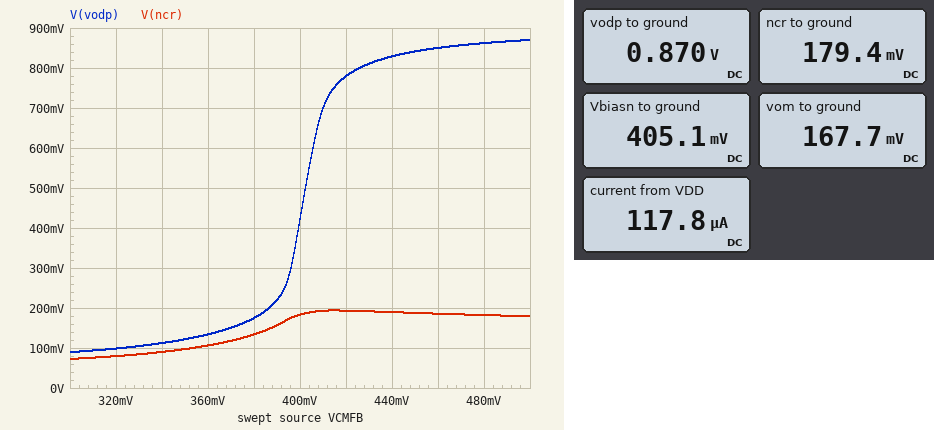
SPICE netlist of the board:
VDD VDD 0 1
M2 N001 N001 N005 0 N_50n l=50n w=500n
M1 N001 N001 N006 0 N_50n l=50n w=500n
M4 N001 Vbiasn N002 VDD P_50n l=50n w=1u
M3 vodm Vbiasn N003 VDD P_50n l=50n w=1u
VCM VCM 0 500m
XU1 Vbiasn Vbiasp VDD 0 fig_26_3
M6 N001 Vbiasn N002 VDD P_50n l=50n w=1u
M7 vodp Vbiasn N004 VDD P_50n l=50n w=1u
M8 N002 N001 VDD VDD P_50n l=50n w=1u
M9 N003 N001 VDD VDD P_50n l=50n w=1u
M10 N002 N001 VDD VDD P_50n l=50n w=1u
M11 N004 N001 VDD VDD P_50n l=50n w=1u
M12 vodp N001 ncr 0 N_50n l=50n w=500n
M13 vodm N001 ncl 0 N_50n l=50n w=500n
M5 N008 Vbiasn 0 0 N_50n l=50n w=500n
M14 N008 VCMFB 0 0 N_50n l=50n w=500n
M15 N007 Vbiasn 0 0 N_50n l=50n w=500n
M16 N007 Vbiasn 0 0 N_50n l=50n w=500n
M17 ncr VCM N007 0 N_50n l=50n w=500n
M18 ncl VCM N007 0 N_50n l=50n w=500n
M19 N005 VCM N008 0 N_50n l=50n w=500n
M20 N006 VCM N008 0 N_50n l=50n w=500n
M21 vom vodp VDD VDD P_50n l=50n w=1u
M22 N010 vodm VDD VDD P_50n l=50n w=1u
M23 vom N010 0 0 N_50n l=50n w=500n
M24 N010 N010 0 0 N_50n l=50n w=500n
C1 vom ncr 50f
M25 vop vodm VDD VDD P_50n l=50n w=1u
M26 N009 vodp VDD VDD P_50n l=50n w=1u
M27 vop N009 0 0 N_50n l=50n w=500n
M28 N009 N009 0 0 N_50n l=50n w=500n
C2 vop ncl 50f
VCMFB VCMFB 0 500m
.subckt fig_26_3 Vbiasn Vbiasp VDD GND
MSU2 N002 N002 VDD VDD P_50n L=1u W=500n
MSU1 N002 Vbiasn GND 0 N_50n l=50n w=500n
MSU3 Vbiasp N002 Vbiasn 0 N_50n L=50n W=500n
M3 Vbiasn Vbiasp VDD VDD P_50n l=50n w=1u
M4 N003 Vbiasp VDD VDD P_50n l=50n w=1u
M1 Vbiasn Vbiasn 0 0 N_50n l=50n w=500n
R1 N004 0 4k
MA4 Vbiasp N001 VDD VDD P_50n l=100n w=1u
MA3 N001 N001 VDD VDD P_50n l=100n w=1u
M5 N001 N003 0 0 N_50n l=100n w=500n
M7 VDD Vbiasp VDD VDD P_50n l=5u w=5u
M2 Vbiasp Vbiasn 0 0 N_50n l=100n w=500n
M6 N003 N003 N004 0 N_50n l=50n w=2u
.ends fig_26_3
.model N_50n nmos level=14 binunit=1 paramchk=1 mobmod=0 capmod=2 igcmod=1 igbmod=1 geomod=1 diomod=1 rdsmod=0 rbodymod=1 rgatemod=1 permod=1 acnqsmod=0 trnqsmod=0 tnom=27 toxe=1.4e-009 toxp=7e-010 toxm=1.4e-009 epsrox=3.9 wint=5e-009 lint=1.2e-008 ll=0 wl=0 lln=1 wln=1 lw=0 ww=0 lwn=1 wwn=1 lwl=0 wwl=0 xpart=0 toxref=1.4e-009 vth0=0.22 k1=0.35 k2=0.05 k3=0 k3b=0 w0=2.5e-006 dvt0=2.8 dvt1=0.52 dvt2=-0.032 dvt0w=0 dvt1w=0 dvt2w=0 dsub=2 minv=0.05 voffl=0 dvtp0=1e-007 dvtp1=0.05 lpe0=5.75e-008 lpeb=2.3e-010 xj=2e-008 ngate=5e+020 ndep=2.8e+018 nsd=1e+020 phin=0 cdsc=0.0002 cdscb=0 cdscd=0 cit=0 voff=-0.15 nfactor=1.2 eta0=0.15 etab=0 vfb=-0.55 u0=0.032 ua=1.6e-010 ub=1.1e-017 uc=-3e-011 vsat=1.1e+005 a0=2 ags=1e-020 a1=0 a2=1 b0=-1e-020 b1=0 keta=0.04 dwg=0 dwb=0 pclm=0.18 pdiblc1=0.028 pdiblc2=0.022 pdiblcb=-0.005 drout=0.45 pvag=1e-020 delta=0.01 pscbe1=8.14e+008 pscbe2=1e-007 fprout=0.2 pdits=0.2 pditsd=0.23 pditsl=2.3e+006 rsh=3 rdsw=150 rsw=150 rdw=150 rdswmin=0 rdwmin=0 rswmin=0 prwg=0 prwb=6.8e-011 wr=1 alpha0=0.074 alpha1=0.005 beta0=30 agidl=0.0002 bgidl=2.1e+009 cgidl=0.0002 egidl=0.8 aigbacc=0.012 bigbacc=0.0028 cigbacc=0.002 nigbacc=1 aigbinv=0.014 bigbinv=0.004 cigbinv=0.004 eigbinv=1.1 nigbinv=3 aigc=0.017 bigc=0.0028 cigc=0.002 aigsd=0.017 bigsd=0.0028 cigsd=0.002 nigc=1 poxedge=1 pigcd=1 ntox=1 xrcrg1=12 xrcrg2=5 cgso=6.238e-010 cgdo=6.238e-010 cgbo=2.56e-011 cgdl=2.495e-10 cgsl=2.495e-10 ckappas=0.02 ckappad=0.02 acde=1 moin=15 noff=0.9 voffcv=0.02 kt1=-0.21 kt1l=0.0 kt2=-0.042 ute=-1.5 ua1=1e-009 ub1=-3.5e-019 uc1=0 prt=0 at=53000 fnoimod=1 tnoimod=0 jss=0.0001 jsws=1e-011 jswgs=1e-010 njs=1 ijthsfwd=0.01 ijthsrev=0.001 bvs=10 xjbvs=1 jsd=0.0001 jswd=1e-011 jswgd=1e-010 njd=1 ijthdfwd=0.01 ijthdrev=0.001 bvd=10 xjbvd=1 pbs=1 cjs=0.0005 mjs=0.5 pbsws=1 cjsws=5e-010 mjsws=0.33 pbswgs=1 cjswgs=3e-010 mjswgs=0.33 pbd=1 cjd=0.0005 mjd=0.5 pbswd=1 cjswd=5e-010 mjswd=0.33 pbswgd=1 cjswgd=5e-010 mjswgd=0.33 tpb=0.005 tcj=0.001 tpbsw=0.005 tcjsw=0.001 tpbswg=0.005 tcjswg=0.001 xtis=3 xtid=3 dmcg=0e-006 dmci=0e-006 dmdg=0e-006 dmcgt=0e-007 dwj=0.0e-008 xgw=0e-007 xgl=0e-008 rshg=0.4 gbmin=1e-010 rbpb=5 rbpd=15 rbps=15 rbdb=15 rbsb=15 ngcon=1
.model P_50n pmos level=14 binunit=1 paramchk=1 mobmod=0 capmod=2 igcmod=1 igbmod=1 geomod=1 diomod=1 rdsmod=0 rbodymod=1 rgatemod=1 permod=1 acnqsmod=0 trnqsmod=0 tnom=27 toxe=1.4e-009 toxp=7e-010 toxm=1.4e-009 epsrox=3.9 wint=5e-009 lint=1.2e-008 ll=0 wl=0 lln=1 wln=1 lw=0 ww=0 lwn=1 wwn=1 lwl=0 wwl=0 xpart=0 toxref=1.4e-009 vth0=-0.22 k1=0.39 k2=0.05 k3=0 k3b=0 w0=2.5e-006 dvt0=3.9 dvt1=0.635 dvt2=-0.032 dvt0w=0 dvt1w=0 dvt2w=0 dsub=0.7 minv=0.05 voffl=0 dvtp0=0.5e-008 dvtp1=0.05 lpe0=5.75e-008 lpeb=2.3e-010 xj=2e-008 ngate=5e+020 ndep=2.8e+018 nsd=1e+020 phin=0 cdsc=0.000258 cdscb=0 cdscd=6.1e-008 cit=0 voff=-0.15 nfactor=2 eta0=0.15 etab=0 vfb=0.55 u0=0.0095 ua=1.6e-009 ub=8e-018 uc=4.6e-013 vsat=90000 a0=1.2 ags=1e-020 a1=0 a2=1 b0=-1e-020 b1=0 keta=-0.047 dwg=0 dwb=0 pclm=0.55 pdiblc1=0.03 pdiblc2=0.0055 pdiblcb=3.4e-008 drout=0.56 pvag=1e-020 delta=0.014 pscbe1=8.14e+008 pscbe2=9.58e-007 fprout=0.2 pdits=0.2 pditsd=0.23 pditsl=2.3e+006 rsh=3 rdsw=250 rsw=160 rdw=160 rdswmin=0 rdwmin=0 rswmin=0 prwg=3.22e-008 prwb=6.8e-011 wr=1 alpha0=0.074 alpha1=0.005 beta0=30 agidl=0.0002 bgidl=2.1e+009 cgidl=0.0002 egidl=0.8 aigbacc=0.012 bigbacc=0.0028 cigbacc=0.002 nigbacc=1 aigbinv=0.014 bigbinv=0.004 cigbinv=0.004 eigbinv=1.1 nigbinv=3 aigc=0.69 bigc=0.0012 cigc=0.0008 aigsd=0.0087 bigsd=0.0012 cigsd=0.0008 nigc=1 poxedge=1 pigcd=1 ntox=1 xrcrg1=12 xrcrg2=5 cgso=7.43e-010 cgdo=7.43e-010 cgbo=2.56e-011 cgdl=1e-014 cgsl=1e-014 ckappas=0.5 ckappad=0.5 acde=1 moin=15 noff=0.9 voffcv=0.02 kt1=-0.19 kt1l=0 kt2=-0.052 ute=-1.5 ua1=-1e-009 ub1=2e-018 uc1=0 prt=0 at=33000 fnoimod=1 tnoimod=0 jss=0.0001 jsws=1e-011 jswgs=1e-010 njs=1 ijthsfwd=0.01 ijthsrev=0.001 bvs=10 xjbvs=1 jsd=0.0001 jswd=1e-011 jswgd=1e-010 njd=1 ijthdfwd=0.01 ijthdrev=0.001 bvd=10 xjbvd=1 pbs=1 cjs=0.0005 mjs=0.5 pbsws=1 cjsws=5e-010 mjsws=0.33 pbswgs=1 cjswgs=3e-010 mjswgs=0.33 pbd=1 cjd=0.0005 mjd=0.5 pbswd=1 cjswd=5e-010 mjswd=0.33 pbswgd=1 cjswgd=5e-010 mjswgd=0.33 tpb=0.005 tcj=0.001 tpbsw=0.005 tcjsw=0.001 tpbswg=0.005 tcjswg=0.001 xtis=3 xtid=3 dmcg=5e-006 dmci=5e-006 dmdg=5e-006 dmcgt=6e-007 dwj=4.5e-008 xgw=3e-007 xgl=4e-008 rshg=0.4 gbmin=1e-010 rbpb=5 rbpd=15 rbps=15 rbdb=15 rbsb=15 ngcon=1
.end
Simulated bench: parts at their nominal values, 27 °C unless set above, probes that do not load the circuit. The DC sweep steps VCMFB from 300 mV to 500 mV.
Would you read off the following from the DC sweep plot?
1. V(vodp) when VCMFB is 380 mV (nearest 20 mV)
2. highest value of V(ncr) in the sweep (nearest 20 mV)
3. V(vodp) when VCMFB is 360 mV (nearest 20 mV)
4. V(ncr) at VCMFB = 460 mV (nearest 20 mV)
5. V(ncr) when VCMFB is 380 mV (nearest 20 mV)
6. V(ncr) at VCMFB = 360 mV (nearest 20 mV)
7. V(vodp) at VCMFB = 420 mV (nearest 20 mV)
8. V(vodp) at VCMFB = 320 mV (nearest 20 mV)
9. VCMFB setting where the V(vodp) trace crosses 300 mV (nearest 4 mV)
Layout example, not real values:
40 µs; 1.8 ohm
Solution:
180 mV; 200 mV; 140 mV; 180 mV; 140 mV; 100 mV; 780 mV; 100 mV; 396 mV
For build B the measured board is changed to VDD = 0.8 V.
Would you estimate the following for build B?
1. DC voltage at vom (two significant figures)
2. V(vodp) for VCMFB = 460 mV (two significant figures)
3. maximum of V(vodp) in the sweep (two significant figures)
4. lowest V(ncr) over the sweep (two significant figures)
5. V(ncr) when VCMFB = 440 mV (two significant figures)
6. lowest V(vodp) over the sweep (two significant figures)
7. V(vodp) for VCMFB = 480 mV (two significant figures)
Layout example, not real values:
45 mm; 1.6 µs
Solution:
310 mV; 460 mV; 490 mV; 45 mV; 46 mV; 160 mV; 470 mV
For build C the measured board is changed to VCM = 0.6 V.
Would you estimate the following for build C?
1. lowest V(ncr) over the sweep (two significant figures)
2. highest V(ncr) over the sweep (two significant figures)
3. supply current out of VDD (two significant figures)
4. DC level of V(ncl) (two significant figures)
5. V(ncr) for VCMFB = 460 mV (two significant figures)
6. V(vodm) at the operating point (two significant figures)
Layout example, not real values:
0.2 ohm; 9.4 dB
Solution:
70 mV; 180 mV; 130 µA; 160 mV; 170 mV; 870 mV
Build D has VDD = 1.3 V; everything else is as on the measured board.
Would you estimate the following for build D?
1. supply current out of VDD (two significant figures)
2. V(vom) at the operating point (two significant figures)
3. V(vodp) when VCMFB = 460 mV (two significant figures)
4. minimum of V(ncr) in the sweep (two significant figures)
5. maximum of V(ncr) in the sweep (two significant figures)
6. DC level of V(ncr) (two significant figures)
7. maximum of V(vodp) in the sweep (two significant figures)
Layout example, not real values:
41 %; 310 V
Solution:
130 µA; 190 mV; 1.1 V; 94 mV; 470 mV; 460 mV; 1.2 V
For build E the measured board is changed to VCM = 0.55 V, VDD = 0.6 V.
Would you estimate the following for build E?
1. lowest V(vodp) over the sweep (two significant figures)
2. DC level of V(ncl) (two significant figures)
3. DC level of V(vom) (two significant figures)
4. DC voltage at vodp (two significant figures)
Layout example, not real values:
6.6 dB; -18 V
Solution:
200 mV; 2.0 mV; 370 mV; 210 mV
